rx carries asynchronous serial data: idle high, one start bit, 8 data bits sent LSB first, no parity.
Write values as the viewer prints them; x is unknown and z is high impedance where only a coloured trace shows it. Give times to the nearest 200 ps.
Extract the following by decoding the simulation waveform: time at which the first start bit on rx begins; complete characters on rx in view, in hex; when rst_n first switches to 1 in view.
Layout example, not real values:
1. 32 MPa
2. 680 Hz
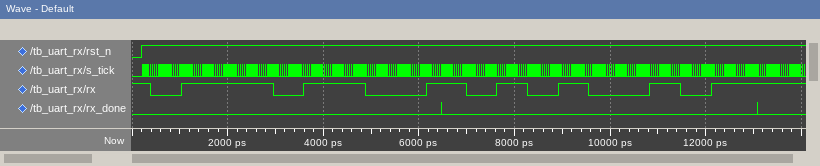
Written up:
1. 400 ps
2. 37, A5
3. 200 ps
